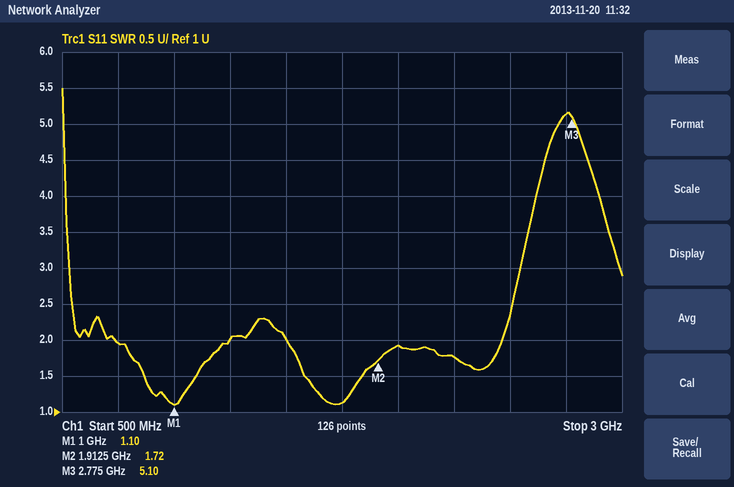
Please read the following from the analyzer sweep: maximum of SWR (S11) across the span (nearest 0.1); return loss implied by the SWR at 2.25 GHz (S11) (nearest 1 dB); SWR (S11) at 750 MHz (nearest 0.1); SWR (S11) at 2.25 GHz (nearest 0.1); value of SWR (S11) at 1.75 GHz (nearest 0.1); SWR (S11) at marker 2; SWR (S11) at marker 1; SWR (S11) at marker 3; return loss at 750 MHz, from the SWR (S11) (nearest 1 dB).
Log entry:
5.5
11 dB
2.0
1.8
1.1
1.72
1.10
5.10
10 dB
